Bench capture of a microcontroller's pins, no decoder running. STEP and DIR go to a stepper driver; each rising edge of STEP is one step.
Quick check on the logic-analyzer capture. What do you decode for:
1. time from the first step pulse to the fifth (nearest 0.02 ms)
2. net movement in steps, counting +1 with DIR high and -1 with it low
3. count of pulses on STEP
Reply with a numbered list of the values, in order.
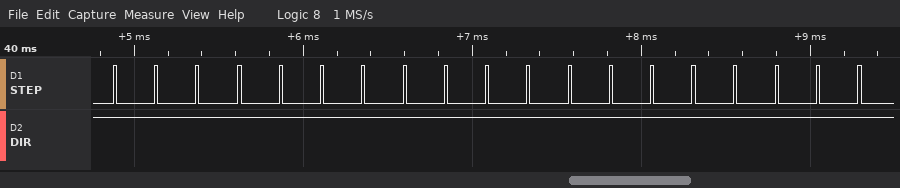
1. 0.98 ms
2. +19
3. 19
